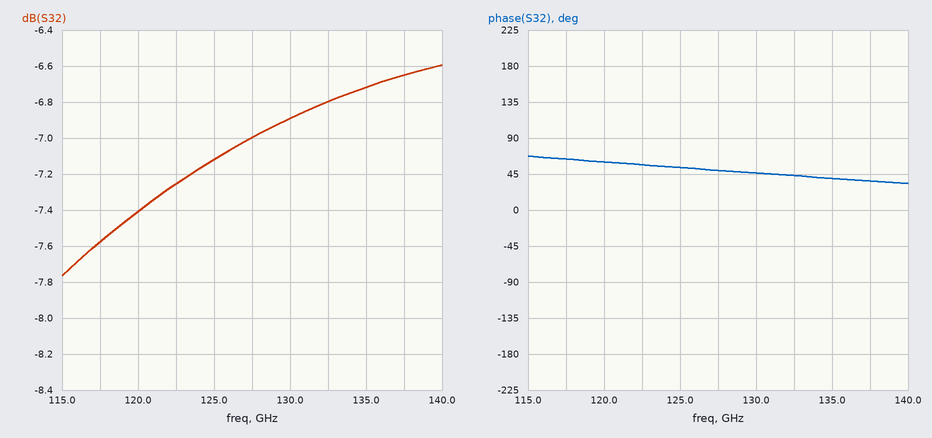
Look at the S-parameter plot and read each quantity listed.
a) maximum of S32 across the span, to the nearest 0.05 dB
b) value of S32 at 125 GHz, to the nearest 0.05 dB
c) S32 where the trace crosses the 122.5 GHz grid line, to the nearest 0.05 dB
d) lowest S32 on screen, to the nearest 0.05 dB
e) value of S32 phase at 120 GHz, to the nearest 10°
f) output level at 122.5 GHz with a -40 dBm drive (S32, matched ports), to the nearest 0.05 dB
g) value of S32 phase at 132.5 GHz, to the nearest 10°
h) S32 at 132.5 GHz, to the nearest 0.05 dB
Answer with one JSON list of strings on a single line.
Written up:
["-6.60 dB", "-7.10 dB", "-7.25 dB", "-7.75 dB", "60°", "-47.25 dBm", "40°", "-6.80 dB"]
